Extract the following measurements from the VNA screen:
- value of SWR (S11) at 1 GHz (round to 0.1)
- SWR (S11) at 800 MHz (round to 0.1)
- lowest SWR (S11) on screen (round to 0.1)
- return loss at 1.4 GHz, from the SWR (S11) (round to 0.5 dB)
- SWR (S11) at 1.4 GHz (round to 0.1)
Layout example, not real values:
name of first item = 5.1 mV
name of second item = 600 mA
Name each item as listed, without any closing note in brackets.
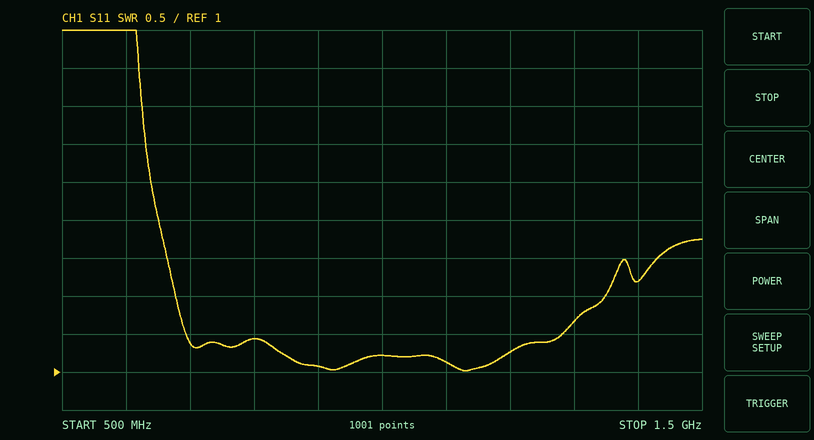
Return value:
value of SWR (S11) at 1 GHz = 1.2
SWR (S11) at 800 MHz = 1.4
lowest SWR (S11) on screen = 1.0
return loss at 1.4 GHz, from the SWR (S11) = 8.5 dB
SWR (S11) at 1.4 GHz = 2.2
